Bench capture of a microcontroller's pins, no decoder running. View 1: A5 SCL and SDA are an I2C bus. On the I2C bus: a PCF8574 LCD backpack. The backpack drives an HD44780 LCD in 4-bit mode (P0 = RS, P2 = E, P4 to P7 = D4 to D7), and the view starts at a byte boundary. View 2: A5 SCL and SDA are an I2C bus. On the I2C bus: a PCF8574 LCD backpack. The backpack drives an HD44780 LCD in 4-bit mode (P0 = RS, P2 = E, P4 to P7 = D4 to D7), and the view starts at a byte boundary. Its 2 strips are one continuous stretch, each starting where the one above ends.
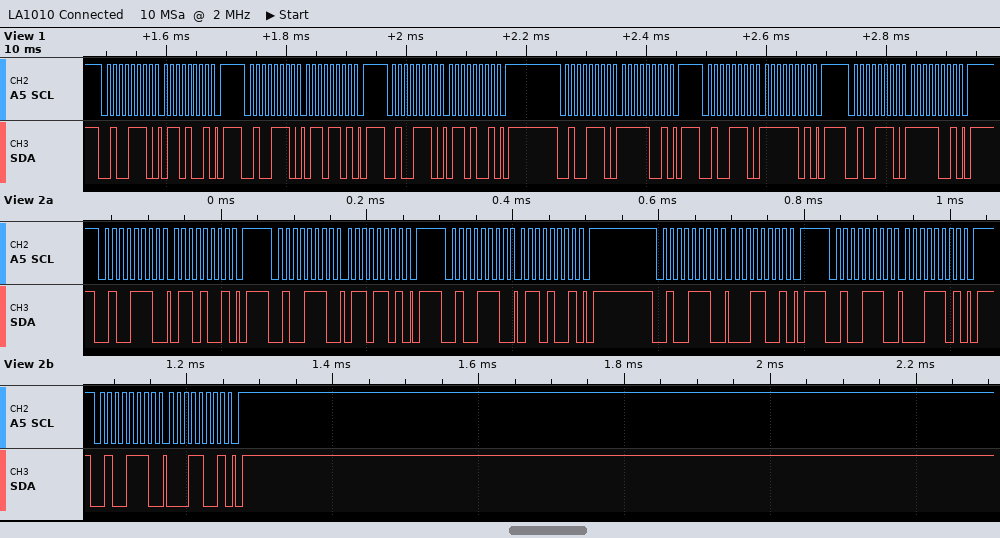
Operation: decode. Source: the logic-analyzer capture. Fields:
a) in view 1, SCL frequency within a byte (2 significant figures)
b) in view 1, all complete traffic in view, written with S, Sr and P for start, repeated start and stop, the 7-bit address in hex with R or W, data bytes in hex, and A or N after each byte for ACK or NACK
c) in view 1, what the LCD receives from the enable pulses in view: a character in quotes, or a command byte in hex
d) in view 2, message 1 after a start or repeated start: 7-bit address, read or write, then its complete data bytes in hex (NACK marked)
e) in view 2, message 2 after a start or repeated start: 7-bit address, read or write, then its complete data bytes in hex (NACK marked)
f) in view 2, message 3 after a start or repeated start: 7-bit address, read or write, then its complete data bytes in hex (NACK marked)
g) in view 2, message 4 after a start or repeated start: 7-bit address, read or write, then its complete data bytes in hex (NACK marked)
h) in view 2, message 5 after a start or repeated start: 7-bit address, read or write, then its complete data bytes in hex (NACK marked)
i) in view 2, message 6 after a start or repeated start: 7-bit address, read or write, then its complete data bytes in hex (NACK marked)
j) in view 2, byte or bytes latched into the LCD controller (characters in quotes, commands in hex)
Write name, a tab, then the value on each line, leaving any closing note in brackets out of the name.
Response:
in view 1, SCL frequency within a byte	100 kHz
in view 1, all complete traffic in view, written with S, Sr and P for start, repeated start and stop, the 7-bit address in hex with R or W, data bytes in hex, and A or N after each byte for ACK or NACK	S 27W A 69 A P S 27W A 6D A P S 27W A 69 A P S 27W A F9 A P S 27W A FD A P S 27W A F9 A P
in view 1, what the LCD receives from the enable pulses in view: a character in quotes, or a command byte in hex	'o'
in view 2, message 1 after a start or repeated start: 7-bit address, read or write, then its complete data bytes in hex	0x27 write: 69
in view 2, message 2 after a start or repeated start: 7-bit address, read or write, then its complete data bytes in hex	0x27 write: 6D
in view 2, message 3 after a start or repeated start: 7-bit address, read or write, then its complete data bytes in hex	0x27 write: 69
in view 2, message 4 after a start or repeated start: 7-bit address, read or write, then its complete data bytes in hex	0x27 write: 19
in view 2, message 5 after a start or repeated start: 7-bit address, read or write, then its complete data bytes in hex	0x27 write: 1D
in view 2, message 6 after a start or repeated start: 7-bit address, read or write, then its complete data bytes in hex	0x27 write: 19
in view 2, byte or bytes latched into the LCD controller	'a'
